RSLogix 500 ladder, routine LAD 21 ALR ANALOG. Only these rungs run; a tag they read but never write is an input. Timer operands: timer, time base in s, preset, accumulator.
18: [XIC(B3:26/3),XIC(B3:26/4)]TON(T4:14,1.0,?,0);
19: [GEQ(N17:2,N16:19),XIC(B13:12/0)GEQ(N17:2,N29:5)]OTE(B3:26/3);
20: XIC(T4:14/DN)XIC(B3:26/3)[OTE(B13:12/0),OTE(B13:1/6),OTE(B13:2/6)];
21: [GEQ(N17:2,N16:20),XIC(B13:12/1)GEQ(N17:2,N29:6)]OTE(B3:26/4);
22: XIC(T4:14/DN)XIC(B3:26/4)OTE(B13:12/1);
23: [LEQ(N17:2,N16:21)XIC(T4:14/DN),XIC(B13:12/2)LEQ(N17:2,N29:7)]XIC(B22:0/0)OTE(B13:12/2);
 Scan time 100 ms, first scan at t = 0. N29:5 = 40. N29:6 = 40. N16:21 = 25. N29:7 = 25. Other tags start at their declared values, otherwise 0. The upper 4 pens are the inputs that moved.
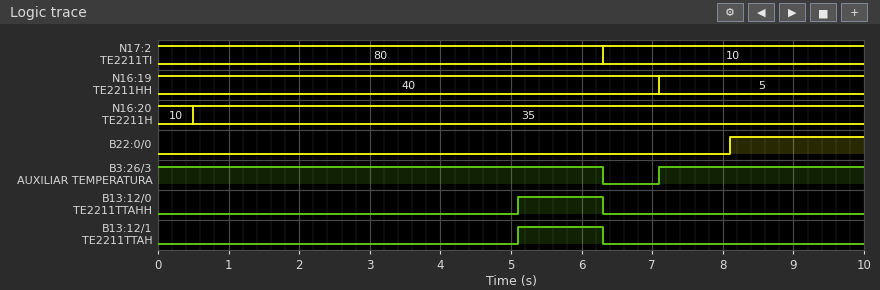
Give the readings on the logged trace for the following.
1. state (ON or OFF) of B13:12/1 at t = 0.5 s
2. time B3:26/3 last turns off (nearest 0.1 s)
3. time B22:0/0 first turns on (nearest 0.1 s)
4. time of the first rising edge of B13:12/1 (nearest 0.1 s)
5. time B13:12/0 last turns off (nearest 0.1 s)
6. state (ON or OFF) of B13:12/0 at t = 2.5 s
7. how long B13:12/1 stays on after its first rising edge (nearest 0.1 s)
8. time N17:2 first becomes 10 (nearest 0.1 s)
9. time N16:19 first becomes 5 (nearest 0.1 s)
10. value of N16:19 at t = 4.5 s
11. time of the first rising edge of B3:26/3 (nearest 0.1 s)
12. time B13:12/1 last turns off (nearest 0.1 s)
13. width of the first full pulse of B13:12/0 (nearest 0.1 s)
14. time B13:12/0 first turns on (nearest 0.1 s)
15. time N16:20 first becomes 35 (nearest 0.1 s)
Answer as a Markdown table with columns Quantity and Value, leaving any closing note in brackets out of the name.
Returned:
| Quantity | Value |
|---|---|
| state (ON or OFF) of B13:12/1 at t = 0.5 s | OFF |
| time B3:26/3 last turns off | 6.3 s |
| time B22:0/0 first turns on | 8.1 s |
| time of the first rising edge of B13:12/1 | 5.1 s |
| time B13:12/0 last turns off | 6.3 s |
| state (ON or OFF) of B13:12/0 at t = 2.5 s | OFF |
| how long B13:12/1 stays on after its first rising edge | 1.2 s |
| time N17:2 first becomes 10 | 6.3 s |
| time N16:19 first becomes 5 | 7.1 s |
| value of N16:19 at t = 4.5 s | 40 |
| time of the first rising edge of B3:26/3 | 7.1 s |
| time B13:12/1 last turns off | 6.3 s |
| width of the first full pulse of B13:12/0 | 1.2 s |
| time B13:12/0 first turns on | 5.1 s |
| time N16:20 first becomes 35 | 0.5 s |
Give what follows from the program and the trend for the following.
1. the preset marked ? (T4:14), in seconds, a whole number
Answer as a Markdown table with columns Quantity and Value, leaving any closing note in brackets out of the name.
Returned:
| Quantity | Value |
|---|---|
| the preset marked ? (T4:14), in seconds, a whole number | 5 s |
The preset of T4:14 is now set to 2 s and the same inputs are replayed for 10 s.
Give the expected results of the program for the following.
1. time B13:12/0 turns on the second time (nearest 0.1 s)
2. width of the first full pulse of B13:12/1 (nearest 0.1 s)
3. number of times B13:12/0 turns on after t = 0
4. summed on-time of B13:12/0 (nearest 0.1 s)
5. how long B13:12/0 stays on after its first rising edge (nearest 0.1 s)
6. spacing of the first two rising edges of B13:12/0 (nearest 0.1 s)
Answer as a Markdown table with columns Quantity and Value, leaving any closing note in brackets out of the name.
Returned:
| Quantity | Value |
|---|---|
| time B13:12/0 turns on the second time | 9.2 s |
| width of the first full pulse of B13:12/1 | 4.2 s |
| number of times B13:12/0 turns on after t = 0 | 2 |
| summed on-time of B13:12/0 | 5.0 s |
| how long B13:12/0 stays on after its first rising edge | 4.2 s |
| spacing of the first two rising edges of B13:12/0 | 7.1 s |
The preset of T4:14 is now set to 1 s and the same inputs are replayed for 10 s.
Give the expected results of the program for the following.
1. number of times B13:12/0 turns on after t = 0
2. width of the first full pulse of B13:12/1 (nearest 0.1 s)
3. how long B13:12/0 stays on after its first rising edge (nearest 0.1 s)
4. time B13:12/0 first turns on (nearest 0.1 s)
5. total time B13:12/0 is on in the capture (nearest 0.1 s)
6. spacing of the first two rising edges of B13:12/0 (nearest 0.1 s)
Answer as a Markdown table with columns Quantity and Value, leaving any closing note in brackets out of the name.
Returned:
| Quantity | Value |
|---|---|
| number of times B13:12/0 turns on after t = 0 | 2 |
| width of the first full pulse of B13:12/1 | 5.2 s |
| how long B13:12/0 stays on after its first rising edge | 5.2 s |
| time B13:12/0 first turns on | 1.1 s |
| total time B13:12/0 is on in the capture | 7.0 s |
| spacing of the first two rising edges of B13:12/0 | 7.1 s |
